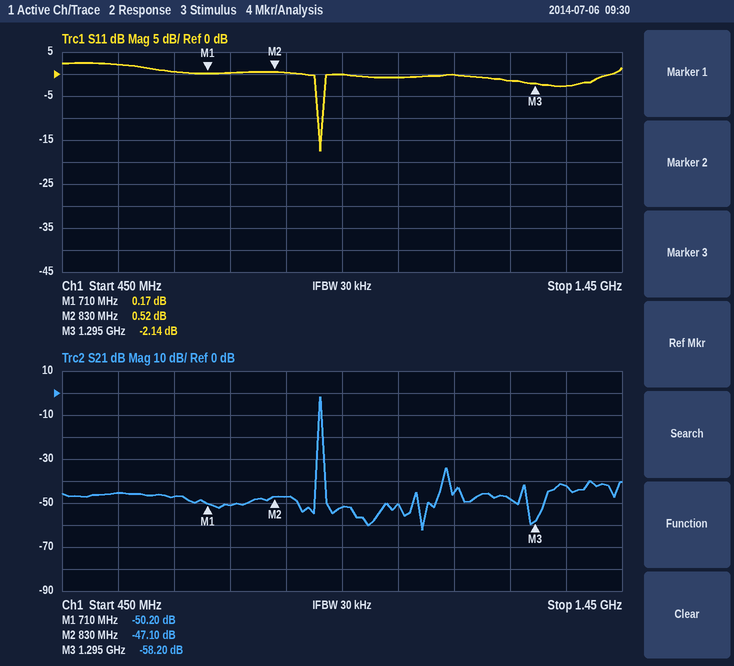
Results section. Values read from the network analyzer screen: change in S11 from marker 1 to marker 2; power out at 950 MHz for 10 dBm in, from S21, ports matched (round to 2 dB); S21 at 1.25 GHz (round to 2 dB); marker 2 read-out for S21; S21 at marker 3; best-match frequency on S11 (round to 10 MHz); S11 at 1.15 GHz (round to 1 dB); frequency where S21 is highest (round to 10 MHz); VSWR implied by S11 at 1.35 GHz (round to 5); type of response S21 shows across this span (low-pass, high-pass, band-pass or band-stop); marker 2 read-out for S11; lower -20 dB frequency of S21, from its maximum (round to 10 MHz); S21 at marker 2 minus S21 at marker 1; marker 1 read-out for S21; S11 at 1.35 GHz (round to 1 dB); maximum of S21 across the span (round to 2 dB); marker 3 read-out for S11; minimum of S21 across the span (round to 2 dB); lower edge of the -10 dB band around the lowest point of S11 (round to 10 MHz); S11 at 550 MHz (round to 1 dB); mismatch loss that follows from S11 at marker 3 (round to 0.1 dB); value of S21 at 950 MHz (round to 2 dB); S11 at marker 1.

0.35 dB
-42 dBm
-48 dB
-47.10 dB
-58.20 dB
910 MHz
0 dB
910 MHz
5
band-pass
0.52 dB
910 MHz
3.10 dB
-50.20 dB
-3 dB
-2 dB
-2.14 dB
-62 dB
910 MHz
2 dB
4.1 dB
-52 dB
0.17 dB
